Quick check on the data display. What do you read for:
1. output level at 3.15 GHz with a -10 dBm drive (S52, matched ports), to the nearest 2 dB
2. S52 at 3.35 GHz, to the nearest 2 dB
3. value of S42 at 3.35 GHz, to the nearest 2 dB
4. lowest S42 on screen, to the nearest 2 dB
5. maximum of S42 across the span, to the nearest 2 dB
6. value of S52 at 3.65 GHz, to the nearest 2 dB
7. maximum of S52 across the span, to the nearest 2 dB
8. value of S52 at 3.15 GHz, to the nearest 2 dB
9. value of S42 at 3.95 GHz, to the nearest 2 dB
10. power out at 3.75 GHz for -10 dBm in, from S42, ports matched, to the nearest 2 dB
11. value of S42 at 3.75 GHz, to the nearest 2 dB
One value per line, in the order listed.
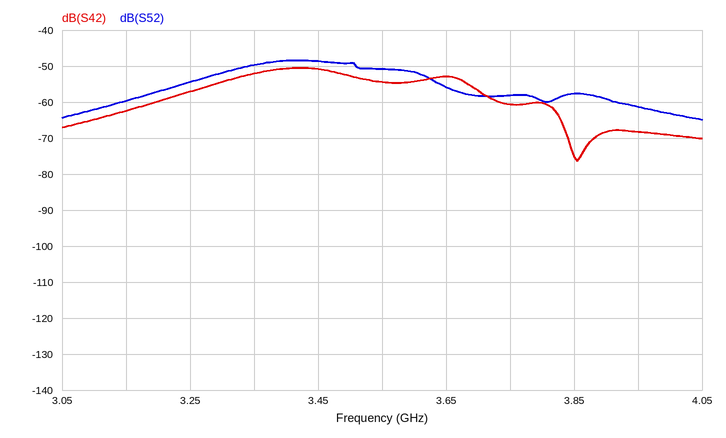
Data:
-70 dBm
-50 dB
-52 dB
-76 dB
-50 dB
-56 dB
-48 dB
-60 dB
-68 dB
-70 dBm
-60 dB
